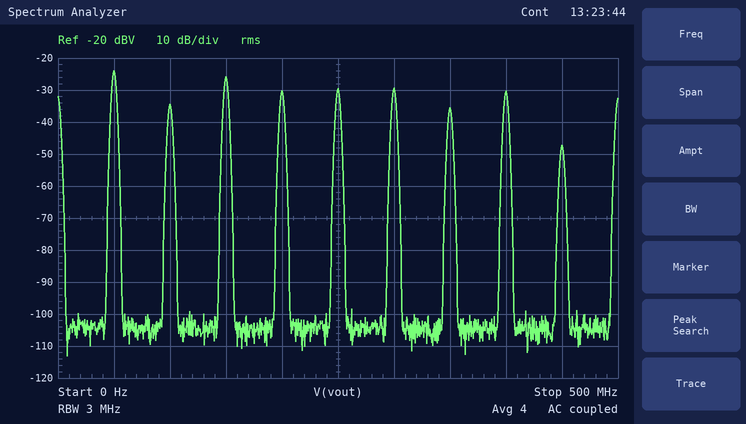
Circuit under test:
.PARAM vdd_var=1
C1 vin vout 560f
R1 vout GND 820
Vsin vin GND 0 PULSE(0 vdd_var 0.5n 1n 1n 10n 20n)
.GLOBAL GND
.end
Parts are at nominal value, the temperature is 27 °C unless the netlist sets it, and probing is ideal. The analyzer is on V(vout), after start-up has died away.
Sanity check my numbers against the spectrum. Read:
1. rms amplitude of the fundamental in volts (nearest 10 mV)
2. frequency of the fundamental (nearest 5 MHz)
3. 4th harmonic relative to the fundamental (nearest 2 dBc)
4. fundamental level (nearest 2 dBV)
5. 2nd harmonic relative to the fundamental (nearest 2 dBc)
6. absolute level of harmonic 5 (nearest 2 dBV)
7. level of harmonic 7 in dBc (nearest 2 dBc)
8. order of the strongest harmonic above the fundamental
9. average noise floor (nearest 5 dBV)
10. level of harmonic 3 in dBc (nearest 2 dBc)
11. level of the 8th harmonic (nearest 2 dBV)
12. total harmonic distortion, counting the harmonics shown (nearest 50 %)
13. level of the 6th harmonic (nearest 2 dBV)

60 mV
50 MHz
-6 dBc
-24 dBV
-10 dBc
-30 dBV
-12 dBc
3
-105 dBV
-2 dBc
-30 dBV
150 %
-30 dBV
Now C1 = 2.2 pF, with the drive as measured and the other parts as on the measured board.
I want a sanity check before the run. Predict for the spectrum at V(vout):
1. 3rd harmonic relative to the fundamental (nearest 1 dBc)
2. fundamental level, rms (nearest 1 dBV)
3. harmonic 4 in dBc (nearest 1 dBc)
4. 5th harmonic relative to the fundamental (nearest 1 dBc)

-6 dBc
-13 dBV
-12 dBc
-12 dBc
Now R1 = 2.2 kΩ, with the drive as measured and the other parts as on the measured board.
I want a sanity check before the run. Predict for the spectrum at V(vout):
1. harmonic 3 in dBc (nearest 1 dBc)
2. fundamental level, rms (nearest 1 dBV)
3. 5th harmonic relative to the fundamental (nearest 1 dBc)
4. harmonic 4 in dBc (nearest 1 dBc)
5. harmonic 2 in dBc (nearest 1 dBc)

-4 dBc
-16 dBV
-10 dBc
-10 dBc
-12 dBc
